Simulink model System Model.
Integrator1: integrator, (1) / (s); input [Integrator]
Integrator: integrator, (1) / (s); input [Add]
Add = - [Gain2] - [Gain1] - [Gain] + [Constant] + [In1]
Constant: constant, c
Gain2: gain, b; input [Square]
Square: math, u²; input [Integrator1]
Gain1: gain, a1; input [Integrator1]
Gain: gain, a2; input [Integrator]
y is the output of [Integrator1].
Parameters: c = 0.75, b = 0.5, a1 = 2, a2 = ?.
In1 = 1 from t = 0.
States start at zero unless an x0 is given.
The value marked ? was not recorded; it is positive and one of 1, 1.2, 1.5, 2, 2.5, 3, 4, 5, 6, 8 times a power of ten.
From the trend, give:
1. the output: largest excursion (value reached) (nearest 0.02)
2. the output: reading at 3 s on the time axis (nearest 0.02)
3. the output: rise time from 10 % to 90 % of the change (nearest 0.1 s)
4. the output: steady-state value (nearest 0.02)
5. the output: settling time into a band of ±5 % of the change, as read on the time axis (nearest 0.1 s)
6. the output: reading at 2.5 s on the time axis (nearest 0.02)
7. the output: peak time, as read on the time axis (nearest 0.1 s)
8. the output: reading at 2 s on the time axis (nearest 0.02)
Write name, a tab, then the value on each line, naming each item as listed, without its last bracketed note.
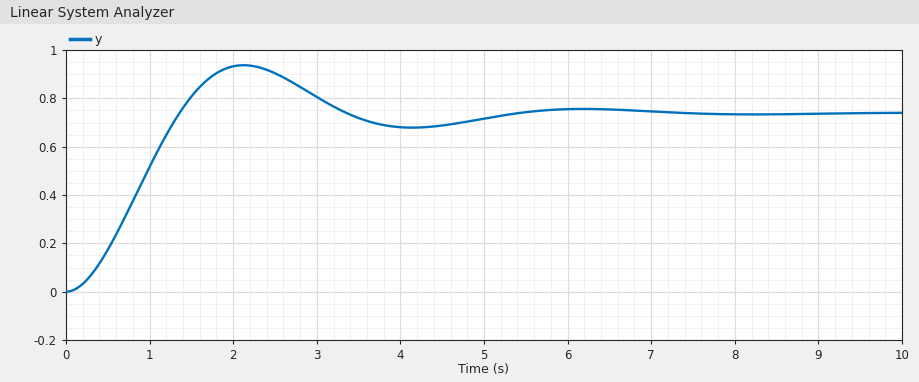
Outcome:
the output: largest excursion (value reached)	0.94
the output: reading at 3 s on the time axis	0.80
the output: rise time from 10 % to 90 % of the change	0.9 s
the output: steady-state value	0.74
the output: settling time into a band of ±5 % of the change, as read on the time axis	4.8 s
the output: reading at 2.5 s on the time axis	0.90
the output: peak time, as read on the time axis	2.1 s
the output: reading at 2 s on the time axis	0.94
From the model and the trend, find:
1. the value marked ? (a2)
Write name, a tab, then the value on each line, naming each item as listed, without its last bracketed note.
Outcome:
the value marked ?	1.2
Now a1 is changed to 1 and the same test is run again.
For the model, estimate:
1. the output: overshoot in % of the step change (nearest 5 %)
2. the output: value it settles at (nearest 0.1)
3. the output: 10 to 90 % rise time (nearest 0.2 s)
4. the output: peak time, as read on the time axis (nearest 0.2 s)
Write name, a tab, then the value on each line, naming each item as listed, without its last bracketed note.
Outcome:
the output: overshoot in % of the step change	20 %
the output: value it settles at	1.1
the output: 10 to 90 % rise time	1.2 s
the output: peak time, as read on the time axis	2.6 s
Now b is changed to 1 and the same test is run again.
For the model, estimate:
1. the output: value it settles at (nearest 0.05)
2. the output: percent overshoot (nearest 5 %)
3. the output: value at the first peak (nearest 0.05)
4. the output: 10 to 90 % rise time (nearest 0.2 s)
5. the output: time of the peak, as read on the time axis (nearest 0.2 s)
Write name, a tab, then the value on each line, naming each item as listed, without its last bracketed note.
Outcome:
the output: value it settles at	0.65
the output: percent overshoot	30 %
the output: value at the first peak	0.85
the output: 10 to 90 % rise time	0.8 s
the output: time of the peak, as read on the time axis	2.0 s
